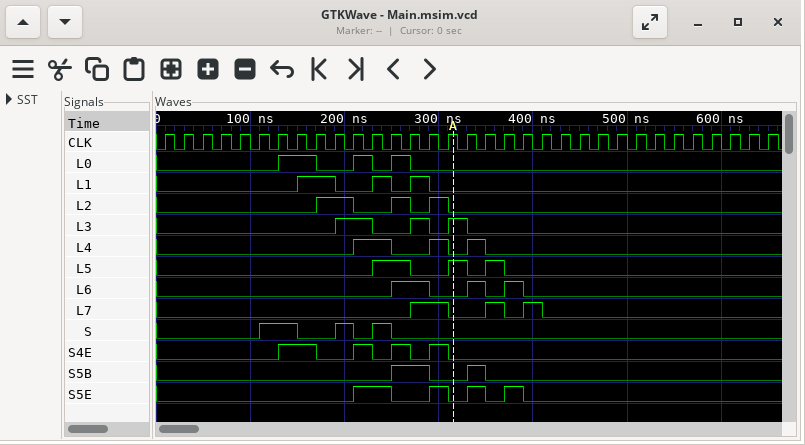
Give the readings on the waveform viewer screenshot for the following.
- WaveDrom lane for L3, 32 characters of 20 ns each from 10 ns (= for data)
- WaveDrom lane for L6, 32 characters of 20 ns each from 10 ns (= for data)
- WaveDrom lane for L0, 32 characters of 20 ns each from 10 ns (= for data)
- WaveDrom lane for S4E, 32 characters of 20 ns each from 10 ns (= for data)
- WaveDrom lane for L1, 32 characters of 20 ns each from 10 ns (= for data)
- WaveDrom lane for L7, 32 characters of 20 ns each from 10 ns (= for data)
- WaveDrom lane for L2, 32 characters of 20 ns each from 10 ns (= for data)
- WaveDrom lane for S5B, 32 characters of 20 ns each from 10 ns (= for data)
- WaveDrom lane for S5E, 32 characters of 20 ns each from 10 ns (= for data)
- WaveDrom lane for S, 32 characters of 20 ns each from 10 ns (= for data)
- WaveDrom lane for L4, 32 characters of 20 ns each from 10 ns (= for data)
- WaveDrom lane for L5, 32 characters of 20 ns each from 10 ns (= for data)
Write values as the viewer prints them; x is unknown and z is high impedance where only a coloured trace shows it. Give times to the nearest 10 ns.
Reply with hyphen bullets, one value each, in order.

- {name: 'L3', wave: '0........1.0.1010...............'}
- {name: 'L6', wave: '0...........1.0.1010............'}
- {name: 'L0', wave: '0.....1.0.1010..................'}
- {name: 'S4E', wave: '0.....1.0.101010................'}
- {name: 'L1', wave: '0......1.0.1010.................'}
- {name: 'L7', wave: '0............1.0.1010...........'}
- {name: 'L2', wave: '0.......1.0.1010................'}
- {name: 'S5B', wave: '0...........1.0.10..............'}
- {name: 'S5E', wave: '0.........1.0.101010............'}
- {name: 'S', wave: '0....1.0.1010...................'}
- {name: 'L4', wave: '0.........1.0.1010..............'}
- {name: 'L5', wave: '0..........1.0.1010.............'}
